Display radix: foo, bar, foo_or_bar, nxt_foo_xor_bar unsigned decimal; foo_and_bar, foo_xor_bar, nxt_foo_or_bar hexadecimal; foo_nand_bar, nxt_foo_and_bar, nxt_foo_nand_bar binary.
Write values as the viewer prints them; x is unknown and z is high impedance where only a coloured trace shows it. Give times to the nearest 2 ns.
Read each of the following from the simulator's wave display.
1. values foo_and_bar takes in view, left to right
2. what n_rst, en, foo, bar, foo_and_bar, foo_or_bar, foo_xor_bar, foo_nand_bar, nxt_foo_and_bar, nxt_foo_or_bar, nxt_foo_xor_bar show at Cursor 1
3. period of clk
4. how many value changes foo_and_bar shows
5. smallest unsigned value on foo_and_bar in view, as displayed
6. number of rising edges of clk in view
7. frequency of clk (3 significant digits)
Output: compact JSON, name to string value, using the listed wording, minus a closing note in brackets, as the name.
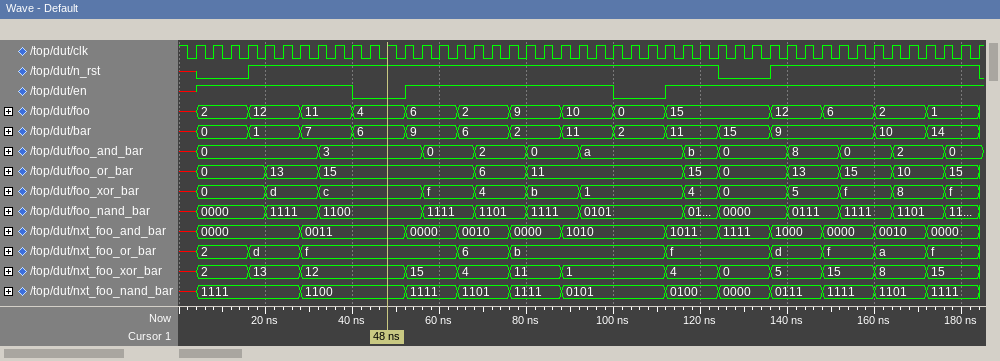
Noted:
{"values foo_and_bar takes in view, left to right": "x, 0, 3, 0, 2, 0, a, b, 0, 8, 0, 2, 0", "what n_rst, en, foo, bar, foo_and_bar, foo_or_bar, foo_xor_bar, foo_nand_bar, nxt_foo_and_bar, nxt_foo_or_bar, nxt_foo_xor_bar show at Cursor 1": "n_rst=1, en=0, foo=4, bar=6, foo_and_bar=3, foo_or_bar=15, foo_xor_bar=c, foo_nand_bar=1100, nxt_foo_and_bar=0011, nxt_foo_or_bar=f, nxt_foo_xor_bar=12", "period of clk": "4 ns", "how many value changes foo_and_bar shows": "12", "smallest unsigned value on foo_and_bar in view, as displayed": "0", "number of rising edges of clk in view": "46", "frequency of clk": "250 MHz"}
